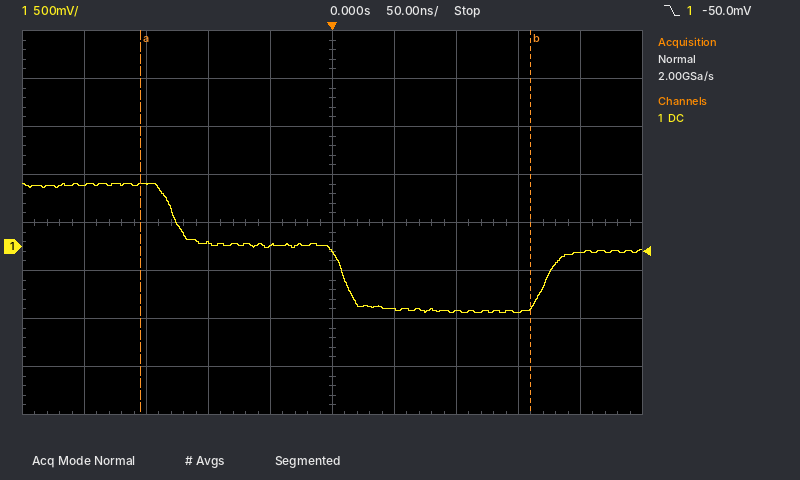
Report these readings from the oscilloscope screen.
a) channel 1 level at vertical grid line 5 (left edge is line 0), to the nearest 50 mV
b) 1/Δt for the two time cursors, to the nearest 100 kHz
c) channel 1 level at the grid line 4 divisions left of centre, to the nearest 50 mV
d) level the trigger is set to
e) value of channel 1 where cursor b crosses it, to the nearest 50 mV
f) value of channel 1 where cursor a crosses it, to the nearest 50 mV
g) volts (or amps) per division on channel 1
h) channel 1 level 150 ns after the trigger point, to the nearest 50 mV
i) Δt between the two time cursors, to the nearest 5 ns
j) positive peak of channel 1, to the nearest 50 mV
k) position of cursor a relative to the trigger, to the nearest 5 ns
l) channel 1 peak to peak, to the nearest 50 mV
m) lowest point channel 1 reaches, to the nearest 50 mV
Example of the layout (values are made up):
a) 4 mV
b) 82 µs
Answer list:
a) -50 mV
b) 3.2 MHz
c) 650 mV
d) -50.0 mV
e) -650 mV
f) 650 mV
g) 500 mV
h) -700 mV
i) 315 ns
j) 650 mV
k) -155 ns
l) 1.35 V
m) -700 mV
